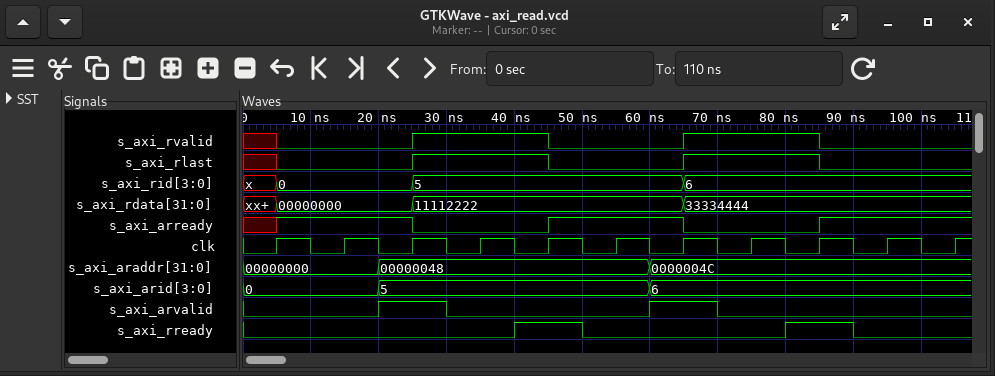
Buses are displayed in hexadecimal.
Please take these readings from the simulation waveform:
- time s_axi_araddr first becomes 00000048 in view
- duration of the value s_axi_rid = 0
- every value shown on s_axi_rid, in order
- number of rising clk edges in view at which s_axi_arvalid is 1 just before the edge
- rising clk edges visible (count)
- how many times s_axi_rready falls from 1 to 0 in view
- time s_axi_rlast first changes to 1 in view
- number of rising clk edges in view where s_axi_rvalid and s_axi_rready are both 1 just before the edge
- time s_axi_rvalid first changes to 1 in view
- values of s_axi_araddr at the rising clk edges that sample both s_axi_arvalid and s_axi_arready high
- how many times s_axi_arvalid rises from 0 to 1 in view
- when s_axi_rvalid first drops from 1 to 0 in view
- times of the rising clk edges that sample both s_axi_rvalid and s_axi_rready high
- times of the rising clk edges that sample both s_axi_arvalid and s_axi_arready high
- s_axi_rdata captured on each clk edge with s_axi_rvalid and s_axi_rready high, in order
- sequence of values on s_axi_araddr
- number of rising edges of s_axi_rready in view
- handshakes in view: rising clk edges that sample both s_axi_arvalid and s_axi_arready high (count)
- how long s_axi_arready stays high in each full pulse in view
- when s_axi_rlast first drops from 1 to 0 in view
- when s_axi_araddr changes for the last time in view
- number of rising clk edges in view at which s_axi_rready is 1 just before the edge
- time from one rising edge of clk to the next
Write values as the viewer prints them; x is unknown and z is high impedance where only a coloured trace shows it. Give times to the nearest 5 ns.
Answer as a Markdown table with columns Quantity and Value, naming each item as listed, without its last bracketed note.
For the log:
| Quantity | Value |
|---|---|
| time s_axi_araddr first becomes 00000048 in view | 20 ns |
| duration of the value s_axi_rid = 0 | 20 ns |
| every value shown on s_axi_rid, in order | x, 0, 5, 6 |
| number of rising clk edges in view at which s_axi_arvalid is 1 just before the edge | 2 |
| rising clk edges visible | 11 |
| how many times s_axi_rready falls from 1 to 0 in view | 2 |
| time s_axi_rlast first changes to 1 in view | 25 ns |
| number of rising clk edges in view where s_axi_rvalid and s_axi_rready are both 1 just before the edge | 2 |
| time s_axi_rvalid first changes to 1 in view | 25 ns |
| values of s_axi_araddr at the rising clk edges that sample both s_axi_arvalid and s_axi_arready high | 00000048, 0000004C |
| how many times s_axi_arvalid rises from 0 to 1 in view | 2 |
| when s_axi_rvalid first drops from 1 to 0 in view | 45 ns |
| times of the rising clk edges that sample both s_axi_rvalid and s_axi_rready high | 45 ns, 85 ns |
| times of the rising clk edges that sample both s_axi_arvalid and s_axi_arready high | 25 ns, 65 ns |
| s_axi_rdata captured on each clk edge with s_axi_rvalid and s_axi_rready high, in order | 11112222, 33334444 |
| sequence of values on s_axi_araddr | 00000000, 00000048, 0000004C |
| number of rising edges of s_axi_rready in view | 2 |
| handshakes in view: rising clk edges that sample both s_axi_arvalid and s_axi_arready high | 2 |
| how long s_axi_arready stays high in each full pulse in view | 20 ns |
| when s_axi_rlast first drops from 1 to 0 in view | 45 ns |
| when s_axi_araddr changes for the last time in view | 60 ns |
| number of rising clk edges in view at which s_axi_rready is 1 just before the edge | 2 |
| time from one rising edge of clk to the next | 10 ns |
